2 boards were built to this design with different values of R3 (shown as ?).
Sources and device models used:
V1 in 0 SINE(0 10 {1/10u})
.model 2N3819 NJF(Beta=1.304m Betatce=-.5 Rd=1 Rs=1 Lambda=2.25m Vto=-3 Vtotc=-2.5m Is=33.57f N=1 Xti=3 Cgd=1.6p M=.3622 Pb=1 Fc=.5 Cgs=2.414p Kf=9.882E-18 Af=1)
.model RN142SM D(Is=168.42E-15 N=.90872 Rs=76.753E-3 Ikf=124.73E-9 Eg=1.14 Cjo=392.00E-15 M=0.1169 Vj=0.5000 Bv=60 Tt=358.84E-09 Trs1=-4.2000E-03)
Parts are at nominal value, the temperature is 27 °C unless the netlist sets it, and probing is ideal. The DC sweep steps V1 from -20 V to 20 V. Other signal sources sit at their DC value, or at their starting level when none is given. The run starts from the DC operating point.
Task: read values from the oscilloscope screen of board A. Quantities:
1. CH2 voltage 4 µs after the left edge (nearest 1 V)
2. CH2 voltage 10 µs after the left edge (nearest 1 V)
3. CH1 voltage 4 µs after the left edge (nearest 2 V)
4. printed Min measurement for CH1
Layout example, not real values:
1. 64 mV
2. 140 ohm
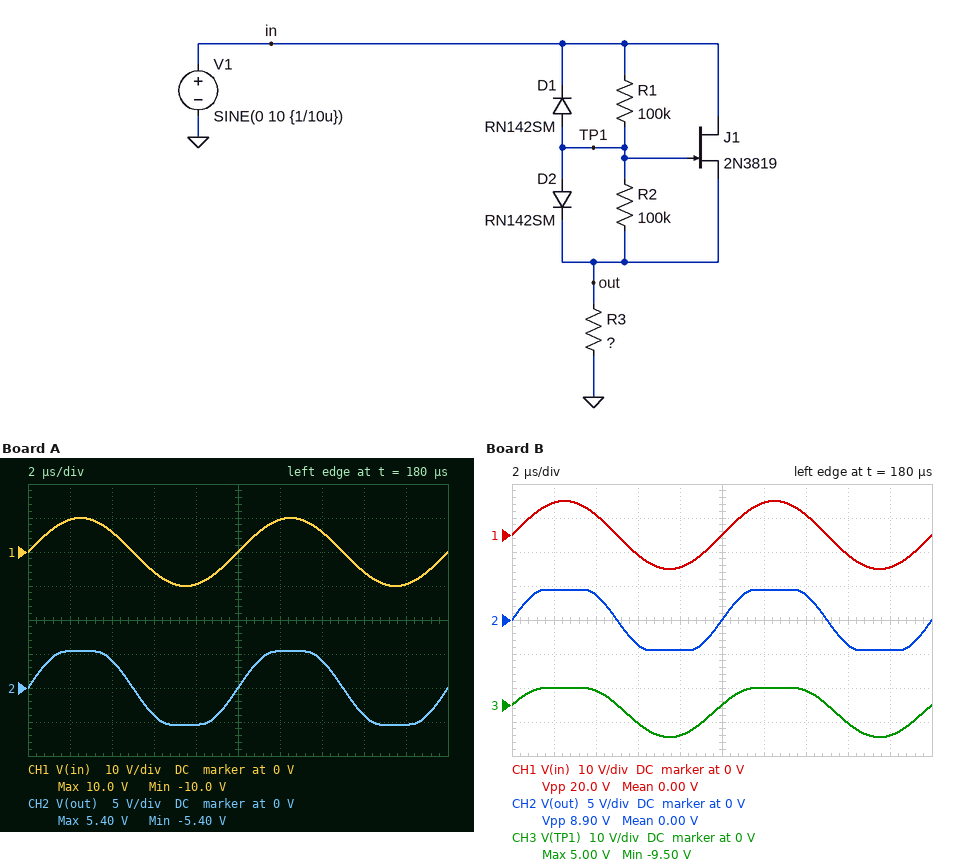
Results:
1. 4 V
2. 0 V
3. 6 V
4. -10.0 V
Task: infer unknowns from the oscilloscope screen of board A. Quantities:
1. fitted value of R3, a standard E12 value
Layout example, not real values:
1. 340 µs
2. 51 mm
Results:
1. 330 Ω
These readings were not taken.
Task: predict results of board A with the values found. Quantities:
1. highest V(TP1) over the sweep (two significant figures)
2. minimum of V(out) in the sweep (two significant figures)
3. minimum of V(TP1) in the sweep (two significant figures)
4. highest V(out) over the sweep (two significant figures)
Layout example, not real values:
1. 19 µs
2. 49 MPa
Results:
1. 6.3 V
2. -5.7 V
3. -19 V
4. 5.7 V
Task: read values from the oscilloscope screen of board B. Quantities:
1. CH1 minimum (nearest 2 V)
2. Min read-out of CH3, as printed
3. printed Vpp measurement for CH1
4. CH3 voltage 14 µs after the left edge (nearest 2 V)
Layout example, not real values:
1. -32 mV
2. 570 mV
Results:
1. -10 V
2. -9.50 V
3. 20.0 V
4. 4 V
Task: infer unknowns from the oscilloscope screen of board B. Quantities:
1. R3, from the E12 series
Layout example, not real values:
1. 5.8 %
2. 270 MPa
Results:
1. 270 Ω
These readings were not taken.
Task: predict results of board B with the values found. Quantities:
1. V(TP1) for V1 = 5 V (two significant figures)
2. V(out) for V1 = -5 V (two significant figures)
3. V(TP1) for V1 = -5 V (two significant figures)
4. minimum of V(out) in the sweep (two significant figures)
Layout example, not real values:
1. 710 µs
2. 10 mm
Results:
1. 3.7 V
2. -3.2 V
3. -4.5 V
4. -4.7 V
